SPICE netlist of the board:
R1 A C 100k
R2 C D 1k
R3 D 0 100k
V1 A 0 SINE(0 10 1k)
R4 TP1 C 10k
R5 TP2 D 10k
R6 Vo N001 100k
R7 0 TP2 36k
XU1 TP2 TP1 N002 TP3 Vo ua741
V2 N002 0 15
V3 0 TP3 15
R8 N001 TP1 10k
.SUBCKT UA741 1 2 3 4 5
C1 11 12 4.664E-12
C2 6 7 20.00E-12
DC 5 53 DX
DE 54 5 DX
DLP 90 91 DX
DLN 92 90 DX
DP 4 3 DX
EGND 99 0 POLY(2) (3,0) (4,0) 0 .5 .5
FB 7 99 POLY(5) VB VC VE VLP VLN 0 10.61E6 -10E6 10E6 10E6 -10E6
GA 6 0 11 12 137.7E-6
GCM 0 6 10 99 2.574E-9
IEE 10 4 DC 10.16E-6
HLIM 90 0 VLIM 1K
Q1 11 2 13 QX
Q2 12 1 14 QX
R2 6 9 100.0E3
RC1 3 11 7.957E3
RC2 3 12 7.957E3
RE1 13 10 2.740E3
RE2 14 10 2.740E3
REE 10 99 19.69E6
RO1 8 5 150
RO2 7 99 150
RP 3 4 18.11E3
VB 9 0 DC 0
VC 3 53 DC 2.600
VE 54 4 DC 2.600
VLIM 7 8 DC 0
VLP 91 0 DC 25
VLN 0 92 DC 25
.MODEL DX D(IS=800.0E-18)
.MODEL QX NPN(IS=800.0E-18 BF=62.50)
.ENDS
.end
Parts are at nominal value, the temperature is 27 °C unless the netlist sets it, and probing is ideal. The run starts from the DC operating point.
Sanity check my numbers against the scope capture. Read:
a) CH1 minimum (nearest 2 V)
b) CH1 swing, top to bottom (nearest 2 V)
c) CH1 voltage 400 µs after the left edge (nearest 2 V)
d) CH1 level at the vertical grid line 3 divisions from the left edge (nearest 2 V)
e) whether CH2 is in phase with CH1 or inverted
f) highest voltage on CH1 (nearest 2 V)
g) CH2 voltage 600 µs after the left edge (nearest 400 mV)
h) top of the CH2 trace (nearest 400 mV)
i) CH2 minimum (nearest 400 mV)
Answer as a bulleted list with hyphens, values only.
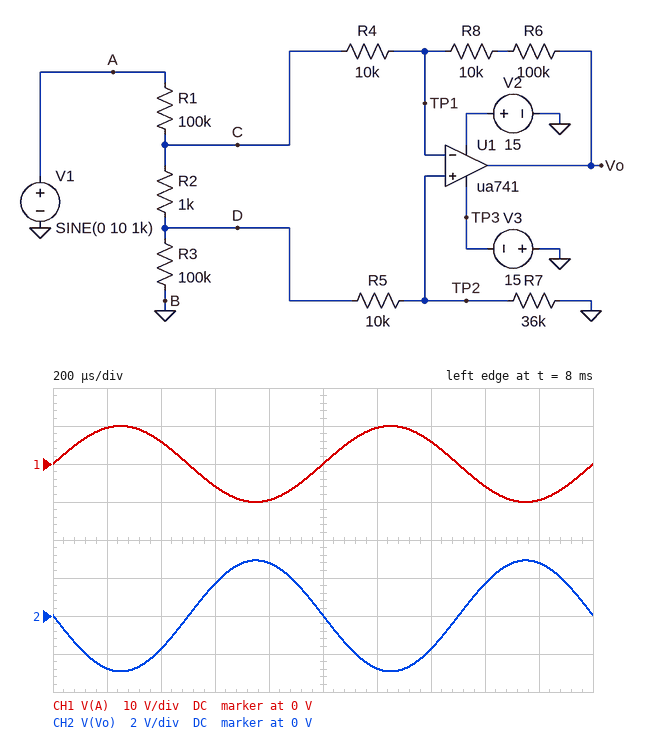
- -10 V
- 20 V
- 6 V
- -6 V
- inverted
- 10 V
- 1.6 V
- 2.8 V
- -2.8 V
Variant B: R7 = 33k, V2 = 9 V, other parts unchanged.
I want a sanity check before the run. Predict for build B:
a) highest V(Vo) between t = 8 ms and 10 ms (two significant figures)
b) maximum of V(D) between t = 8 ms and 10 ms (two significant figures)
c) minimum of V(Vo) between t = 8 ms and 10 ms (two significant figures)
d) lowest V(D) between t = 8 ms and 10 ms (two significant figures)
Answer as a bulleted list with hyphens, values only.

- 3.1 V
- 1.4 V
- -3.1 V
- -1.4 V
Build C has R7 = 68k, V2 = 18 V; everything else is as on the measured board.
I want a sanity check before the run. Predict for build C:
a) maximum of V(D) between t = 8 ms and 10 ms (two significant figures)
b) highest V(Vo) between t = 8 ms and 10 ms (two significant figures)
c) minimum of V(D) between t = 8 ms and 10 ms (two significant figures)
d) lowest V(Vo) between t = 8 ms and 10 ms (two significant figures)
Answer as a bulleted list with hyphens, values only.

- 2.1 V
- 1.6 V
- -2.1 V
- -1.6 V
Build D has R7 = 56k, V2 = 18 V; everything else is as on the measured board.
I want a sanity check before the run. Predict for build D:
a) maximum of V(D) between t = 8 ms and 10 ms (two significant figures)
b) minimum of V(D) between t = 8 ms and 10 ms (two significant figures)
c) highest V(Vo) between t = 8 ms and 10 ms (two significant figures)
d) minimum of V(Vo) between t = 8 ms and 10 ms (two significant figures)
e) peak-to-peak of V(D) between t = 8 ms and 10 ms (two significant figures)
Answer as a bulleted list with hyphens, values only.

- 1.9 V
- -1.9 V
- 2.1 V
- -2.1 V
- 3.8 V
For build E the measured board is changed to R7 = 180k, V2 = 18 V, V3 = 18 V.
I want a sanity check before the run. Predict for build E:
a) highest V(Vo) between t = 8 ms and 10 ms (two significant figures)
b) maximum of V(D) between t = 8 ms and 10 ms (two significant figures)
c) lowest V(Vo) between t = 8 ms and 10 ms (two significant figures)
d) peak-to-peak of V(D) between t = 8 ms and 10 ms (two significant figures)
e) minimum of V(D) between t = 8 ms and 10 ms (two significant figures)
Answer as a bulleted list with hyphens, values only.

- 620 mV
- 3.1 V
- -620 mV
- 6.2 V
- -3.1 V
